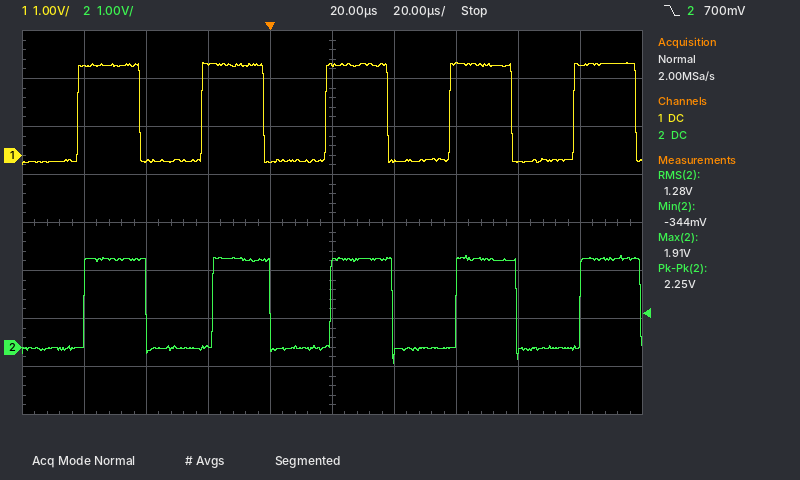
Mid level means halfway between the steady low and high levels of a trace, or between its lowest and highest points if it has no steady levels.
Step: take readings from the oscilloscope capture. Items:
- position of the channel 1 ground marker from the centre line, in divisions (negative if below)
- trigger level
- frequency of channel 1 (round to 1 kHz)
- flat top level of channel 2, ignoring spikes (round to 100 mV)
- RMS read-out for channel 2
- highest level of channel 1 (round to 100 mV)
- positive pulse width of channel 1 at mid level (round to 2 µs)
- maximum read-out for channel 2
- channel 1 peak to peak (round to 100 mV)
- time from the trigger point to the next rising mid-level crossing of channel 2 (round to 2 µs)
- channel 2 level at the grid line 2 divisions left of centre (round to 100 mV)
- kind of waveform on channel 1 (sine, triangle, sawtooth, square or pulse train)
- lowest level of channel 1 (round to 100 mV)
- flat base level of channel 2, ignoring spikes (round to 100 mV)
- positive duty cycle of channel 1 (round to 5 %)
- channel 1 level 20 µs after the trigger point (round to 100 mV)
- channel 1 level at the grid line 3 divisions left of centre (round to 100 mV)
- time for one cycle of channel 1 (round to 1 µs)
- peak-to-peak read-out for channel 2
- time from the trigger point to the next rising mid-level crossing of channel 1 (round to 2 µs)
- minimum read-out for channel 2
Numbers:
+1.4 div
700 mV
25 kHz
1.8 V
1.28 V
1.9 V
20 µs
1.91 V
2.1 V
20 µs
0.0 V
square
-200 mV
0.0 V
50 %
1.9 V
-100 mV
40 µs
2.25 V
18 µs
-344 mV
